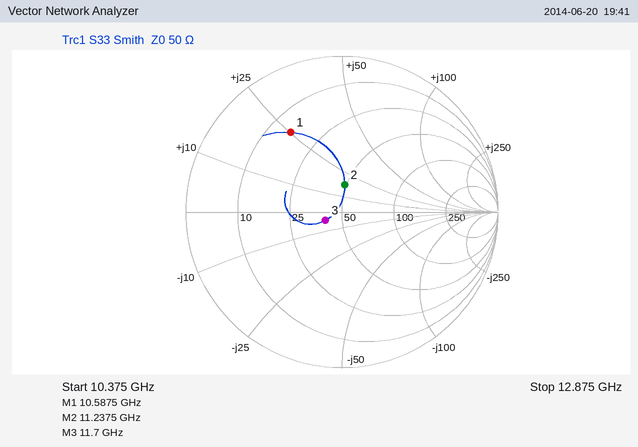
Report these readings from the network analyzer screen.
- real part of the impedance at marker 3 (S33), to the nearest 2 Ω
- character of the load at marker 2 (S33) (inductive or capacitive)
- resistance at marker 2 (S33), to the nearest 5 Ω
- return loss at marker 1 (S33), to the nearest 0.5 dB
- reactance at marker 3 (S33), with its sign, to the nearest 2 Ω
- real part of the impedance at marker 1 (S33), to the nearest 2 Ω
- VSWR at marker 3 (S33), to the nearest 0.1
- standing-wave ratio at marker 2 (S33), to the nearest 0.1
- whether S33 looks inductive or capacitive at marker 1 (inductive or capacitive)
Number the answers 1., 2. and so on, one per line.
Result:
1. 40 Ω
2. inductive
3. 50 Ω
4. 4.5 dB
5. -4 Ω
6. 16 Ω
7. 1.3
8. 1.4
9. inductive
